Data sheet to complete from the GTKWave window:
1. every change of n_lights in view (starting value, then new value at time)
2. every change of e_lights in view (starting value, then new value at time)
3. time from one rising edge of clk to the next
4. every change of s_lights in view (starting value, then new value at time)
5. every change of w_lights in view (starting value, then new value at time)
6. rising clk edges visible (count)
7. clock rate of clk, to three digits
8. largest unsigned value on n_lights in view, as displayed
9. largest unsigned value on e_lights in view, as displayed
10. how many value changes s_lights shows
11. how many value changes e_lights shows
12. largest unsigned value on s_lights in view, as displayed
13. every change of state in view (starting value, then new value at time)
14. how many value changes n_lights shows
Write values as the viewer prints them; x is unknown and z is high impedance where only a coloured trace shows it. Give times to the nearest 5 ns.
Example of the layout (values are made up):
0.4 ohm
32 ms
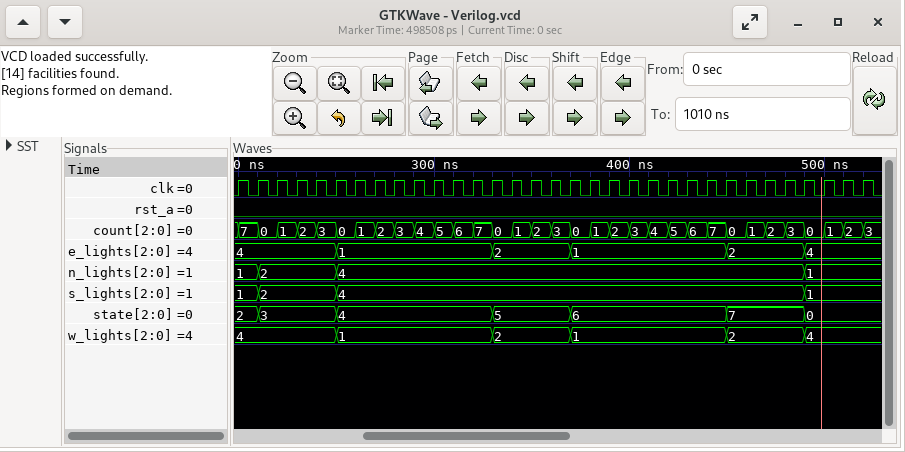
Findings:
1, 2 at 210 ns, 4 at 250 ns, 1 at 490 ns
4, 1 at 250 ns, 2 at 330 ns, 1 at 370 ns, 2 at 450 ns, 4 at 490 ns
10 ns
1, 2 at 210 ns, 4 at 250 ns, 1 at 490 ns
4, 1 at 250 ns, 2 at 330 ns, 1 at 370 ns, 2 at 450 ns, 4 at 490 ns
33
100 MHz
4
4
3
5
4
2, 3 at 210 ns, 4 at 250 ns, 5 at 330 ns, 6 at 370 ns, 7 at 450 ns, 0 at 490 ns
3
